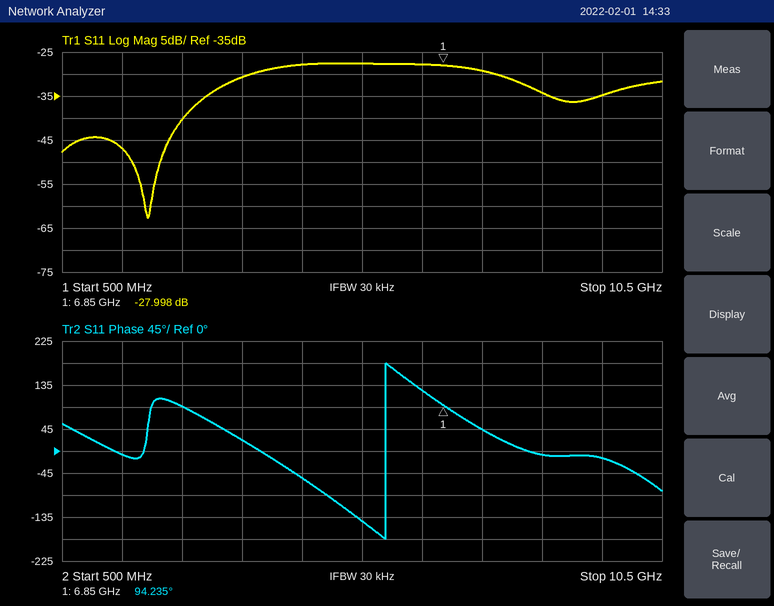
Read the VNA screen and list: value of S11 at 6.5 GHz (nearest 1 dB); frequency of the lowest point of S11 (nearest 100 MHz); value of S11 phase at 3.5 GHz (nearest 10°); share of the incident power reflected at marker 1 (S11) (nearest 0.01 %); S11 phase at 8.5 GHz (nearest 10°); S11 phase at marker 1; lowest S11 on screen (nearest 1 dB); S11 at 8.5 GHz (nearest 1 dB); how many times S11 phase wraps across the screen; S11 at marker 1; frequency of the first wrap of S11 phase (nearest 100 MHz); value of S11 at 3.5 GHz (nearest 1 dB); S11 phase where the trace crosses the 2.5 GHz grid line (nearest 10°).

-28 dB
1.9 GHz
20°
0.16 %
-10°
94.235°
-63 dB
-34 dB
1
-27.998 dB
5.9 GHz
-31 dB
90°
